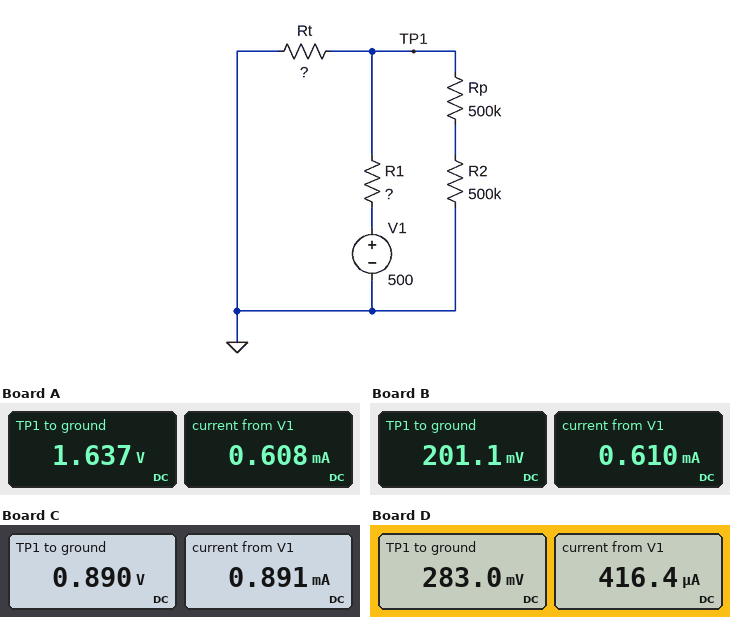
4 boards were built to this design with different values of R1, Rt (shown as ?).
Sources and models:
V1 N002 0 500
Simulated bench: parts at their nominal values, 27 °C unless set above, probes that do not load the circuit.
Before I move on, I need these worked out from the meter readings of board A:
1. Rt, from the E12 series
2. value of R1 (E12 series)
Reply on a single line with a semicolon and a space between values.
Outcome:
2.7 kΩ; 820 kΩ
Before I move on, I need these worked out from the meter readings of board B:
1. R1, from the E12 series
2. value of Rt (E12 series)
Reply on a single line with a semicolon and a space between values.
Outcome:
820 kΩ; 330 Ω
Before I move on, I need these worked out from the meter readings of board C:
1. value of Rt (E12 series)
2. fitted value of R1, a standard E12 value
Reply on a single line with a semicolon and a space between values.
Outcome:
1 kΩ; 560 kΩ
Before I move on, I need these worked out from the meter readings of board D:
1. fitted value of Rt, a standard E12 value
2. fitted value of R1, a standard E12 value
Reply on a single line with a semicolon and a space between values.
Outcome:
680 Ω; 1.2 MΩ
